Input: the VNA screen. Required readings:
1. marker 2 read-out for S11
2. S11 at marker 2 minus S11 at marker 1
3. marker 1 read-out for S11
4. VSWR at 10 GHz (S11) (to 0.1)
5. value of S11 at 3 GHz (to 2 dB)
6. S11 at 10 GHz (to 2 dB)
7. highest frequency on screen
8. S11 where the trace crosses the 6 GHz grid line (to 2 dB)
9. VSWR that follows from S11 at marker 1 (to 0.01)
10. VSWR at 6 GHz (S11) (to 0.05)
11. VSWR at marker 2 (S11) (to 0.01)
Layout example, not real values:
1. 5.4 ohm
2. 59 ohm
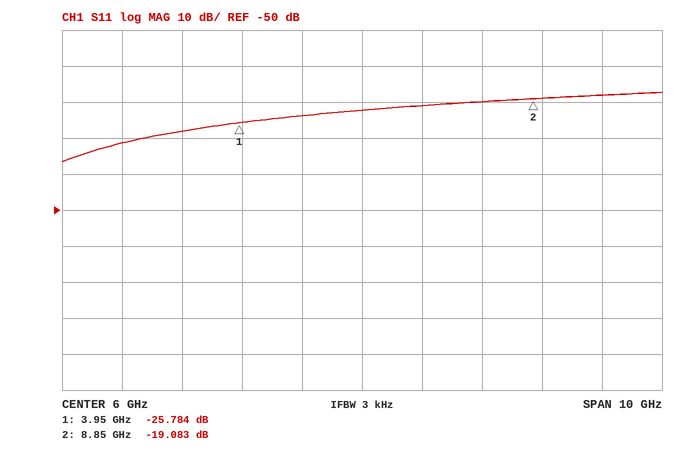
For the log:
1. -19.083 dB
2. 6.701 dB
3. -25.784 dB
4. 1.3
5. -28 dB
6. -18 dB
7. 11 GHz
8. -22 dB
9. 1.11
10. 1.15
11. 1.25
